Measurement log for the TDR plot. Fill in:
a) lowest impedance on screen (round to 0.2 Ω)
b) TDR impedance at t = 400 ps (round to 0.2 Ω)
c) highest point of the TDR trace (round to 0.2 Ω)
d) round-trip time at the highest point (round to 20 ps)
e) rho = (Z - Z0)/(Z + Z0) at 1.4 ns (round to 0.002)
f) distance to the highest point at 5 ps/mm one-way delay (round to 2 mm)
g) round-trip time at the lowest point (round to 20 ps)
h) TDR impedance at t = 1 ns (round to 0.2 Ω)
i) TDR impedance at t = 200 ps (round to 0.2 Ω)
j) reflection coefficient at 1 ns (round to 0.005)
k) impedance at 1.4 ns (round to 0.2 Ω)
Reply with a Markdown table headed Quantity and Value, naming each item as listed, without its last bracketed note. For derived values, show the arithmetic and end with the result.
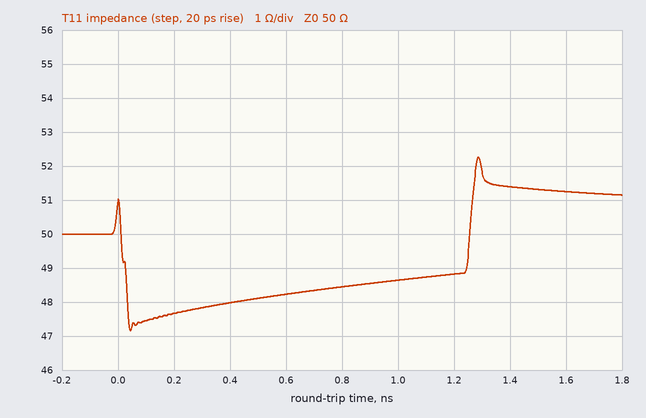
| Quantity | Value |
|---|---|
| lowest impedance on screen | 47.2 Ω |
| TDR impedance at t = 400 ps | 48.0 Ω |
| highest point of the TDR trace | 52.2 Ω |
| round-trip time at the highest point | 1.28 ns |
| rho = (Z - Z0)/(Z + Z0) at 1.4 ns | (51.4 − 50)/(51.4 + 50) ≈ +0.014 |
| distance to the highest point at 5 ps/mm one-way delay | 1.28 ns / 2 / 5 ps/mm ≈ 128 mm |
| round-trip time at the lowest point | 40 ps |
| TDR impedance at t = 1 ns | 48.6 Ω |
| TDR impedance at t = 200 ps | 47.6 Ω |
| reflection coefficient at 1 ns | (48.6 − 50)/(48.6 + 50) ≈ -0.0142, so -0.015 to the nearest 0.005 |
| impedance at 1.4 ns | 51.4 Ω |
